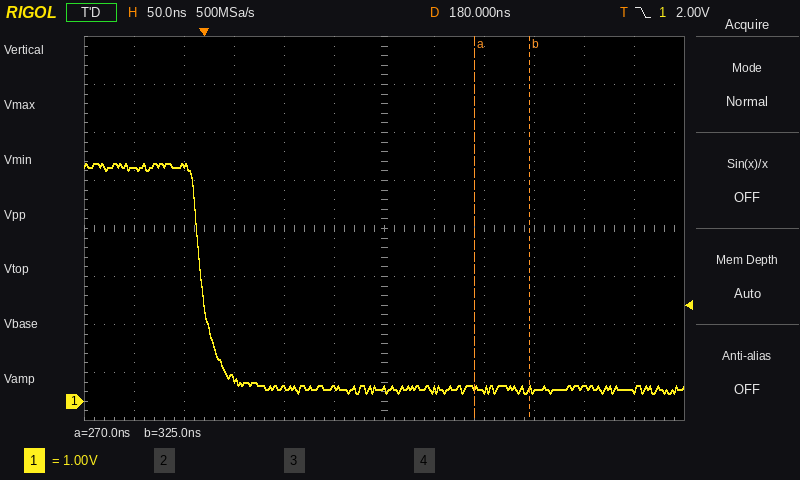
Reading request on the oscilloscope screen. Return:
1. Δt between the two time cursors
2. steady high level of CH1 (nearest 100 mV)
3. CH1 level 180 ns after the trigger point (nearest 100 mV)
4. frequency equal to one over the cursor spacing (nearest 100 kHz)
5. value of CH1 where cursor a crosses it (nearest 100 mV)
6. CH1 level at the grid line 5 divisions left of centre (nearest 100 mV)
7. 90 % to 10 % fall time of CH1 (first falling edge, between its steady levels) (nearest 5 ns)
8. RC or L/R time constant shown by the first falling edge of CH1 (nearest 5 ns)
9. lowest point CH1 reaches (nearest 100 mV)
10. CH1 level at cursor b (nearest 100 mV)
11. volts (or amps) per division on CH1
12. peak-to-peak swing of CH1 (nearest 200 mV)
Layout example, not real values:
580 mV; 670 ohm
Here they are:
55 ns; 4.9 V; 200 mV; 18.2 MHz; 300 mV; 4.9 V; 30 ns; 15 ns; 200 mV; 200 mV; 1 V; 4.8 V
